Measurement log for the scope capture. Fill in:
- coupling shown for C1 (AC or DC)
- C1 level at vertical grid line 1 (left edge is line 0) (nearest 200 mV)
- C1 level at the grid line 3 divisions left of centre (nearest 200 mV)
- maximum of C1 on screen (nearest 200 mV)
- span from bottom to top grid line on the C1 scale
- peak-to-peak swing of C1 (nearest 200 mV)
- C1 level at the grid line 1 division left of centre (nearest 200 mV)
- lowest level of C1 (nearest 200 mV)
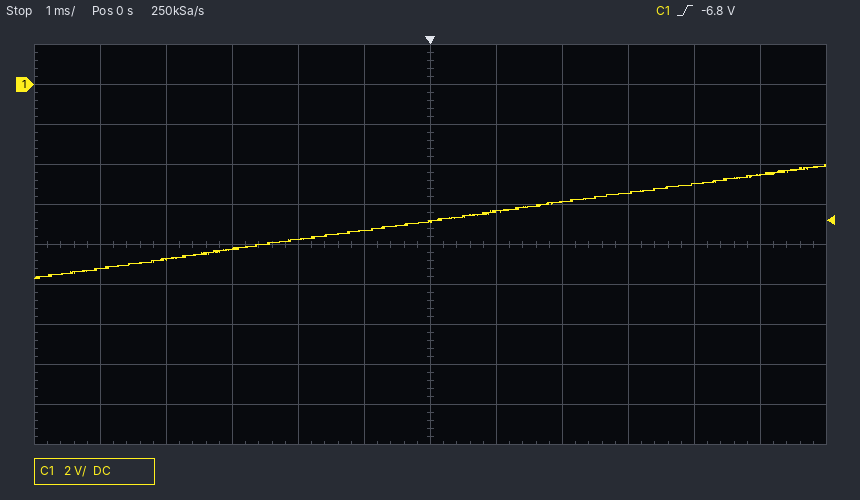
DC
-9.2 V
-8.2 V
-4.0 V
20 V
5.6 V
-7.2 V
-9.6 V
